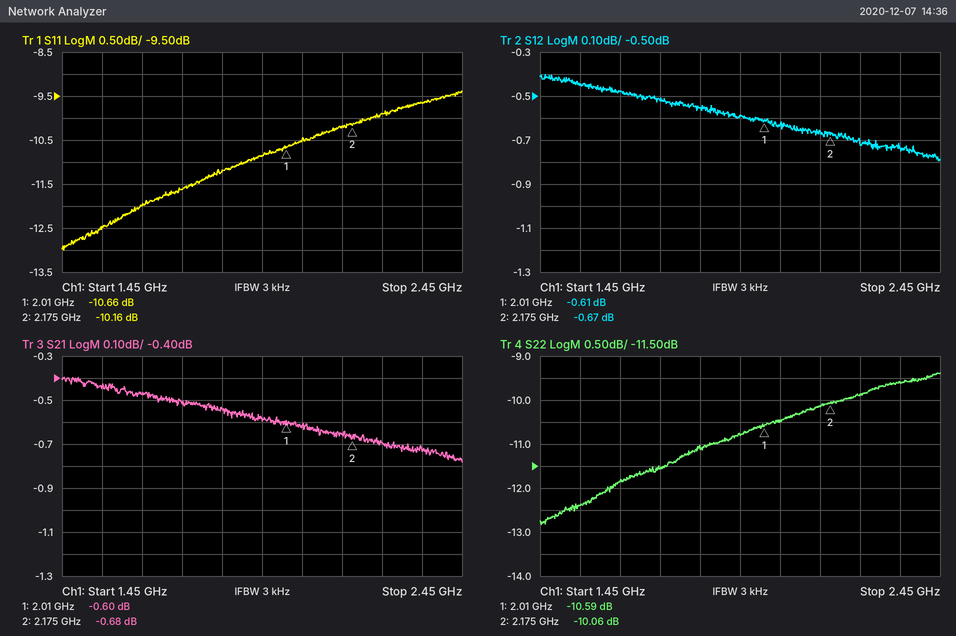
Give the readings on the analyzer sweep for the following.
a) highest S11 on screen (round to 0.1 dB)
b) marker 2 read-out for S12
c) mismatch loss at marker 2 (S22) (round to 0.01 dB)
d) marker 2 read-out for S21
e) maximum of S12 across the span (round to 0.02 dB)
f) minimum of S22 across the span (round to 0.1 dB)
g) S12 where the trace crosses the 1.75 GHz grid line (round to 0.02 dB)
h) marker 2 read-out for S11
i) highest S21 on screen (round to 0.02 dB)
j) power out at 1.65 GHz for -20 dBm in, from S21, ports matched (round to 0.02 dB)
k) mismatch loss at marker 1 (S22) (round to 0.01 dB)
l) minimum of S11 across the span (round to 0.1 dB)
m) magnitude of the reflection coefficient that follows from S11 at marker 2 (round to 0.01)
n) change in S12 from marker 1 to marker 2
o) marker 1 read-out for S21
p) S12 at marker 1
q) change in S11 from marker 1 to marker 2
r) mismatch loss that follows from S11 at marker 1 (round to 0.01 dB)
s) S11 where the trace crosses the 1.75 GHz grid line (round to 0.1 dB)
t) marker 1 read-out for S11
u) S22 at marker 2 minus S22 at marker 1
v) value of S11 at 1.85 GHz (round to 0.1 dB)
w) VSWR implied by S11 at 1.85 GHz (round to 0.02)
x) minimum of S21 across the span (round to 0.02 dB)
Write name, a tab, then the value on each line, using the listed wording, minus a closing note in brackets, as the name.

highest S11 on screen	-9.4 dB
marker 2 read-out for S12	-0.67 dB
mismatch loss at marker 2 (S22)	0.45 dB
marker 2 read-out for S21	-0.68 dB
maximum of S12 across the span	-0.40 dB
minimum of S22 across the span	-12.8 dB
S12 where the trace crosses the 1.75 GHz grid line	-0.52 dB
marker 2 read-out for S11	-10.16 dB
highest S21 on screen	-0.40 dB
power out at 1.65 GHz for -20 dBm in, from S21, ports matched	-20.48 dBm
mismatch loss at marker 1 (S22)	0.40 dB
minimum of S11 across the span	-13.0 dB
magnitude of the reflection coefficient that follows from S11 at marker 2	0.31
change in S12 from marker 1 to marker 2	-0.06 dB
marker 1 read-out for S21	-0.60 dB
S12 at marker 1	-0.61 dB
change in S11 from marker 1 to marker 2	0.50 dB
mismatch loss that follows from S11 at marker 1	0.39 dB
S11 where the trace crosses the 1.75 GHz grid line	-11.6 dB
marker 1 read-out for S11	-10.66 dB
S22 at marker 2 minus S22 at marker 1	0.53 dB
value of S11 at 1.85 GHz	-11.2 dB
VSWR implied by S11 at 1.85 GHz	1.76
minimum of S21 across the span	-0.78 dB
